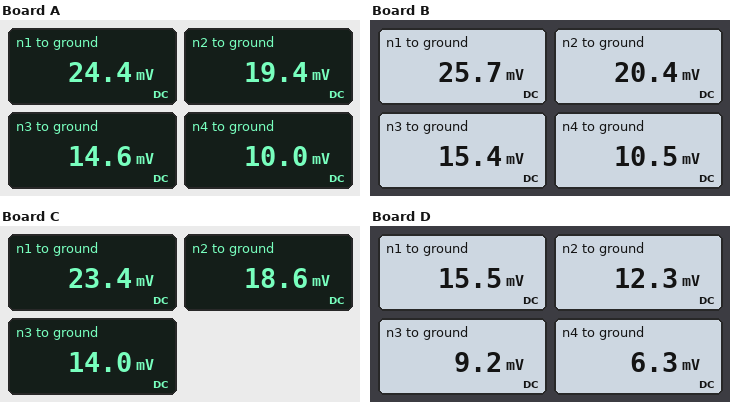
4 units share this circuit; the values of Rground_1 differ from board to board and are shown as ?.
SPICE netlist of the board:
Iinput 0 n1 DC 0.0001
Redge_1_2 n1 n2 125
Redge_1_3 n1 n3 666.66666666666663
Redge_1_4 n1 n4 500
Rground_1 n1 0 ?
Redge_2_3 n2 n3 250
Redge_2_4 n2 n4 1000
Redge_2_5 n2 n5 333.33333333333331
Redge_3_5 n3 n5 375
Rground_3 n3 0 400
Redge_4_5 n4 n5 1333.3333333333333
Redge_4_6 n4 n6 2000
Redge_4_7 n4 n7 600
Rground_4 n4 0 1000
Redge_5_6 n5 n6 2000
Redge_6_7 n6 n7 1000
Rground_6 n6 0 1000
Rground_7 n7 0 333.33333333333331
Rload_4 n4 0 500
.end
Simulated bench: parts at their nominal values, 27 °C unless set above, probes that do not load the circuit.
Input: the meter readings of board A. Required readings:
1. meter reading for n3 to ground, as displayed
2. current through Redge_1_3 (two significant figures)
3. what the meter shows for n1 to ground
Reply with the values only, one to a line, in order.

14.6 mV
15 µA
24.4 mV
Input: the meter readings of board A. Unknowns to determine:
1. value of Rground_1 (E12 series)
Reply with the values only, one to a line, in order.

1.5 kΩ
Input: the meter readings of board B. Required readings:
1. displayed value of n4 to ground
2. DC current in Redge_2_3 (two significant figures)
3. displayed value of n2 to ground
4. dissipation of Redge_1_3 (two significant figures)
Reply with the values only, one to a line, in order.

10.5 mV
20 µA
20.4 mV
160 nW
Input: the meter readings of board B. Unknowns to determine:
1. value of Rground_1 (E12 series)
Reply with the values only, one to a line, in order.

2.2 kΩ
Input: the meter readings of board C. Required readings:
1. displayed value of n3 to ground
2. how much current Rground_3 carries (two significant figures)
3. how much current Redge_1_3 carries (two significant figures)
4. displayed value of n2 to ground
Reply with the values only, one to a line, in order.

14.0 mV
35 µA
14 µA
18.6 mV
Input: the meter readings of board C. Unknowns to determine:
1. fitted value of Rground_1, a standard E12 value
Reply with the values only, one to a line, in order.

1.2 kΩ
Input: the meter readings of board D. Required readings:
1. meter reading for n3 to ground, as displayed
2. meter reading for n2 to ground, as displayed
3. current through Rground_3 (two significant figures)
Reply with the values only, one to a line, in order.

9.2 mV
12.3 mV
23 µA
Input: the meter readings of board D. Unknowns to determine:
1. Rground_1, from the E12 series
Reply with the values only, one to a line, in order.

330 Ω
